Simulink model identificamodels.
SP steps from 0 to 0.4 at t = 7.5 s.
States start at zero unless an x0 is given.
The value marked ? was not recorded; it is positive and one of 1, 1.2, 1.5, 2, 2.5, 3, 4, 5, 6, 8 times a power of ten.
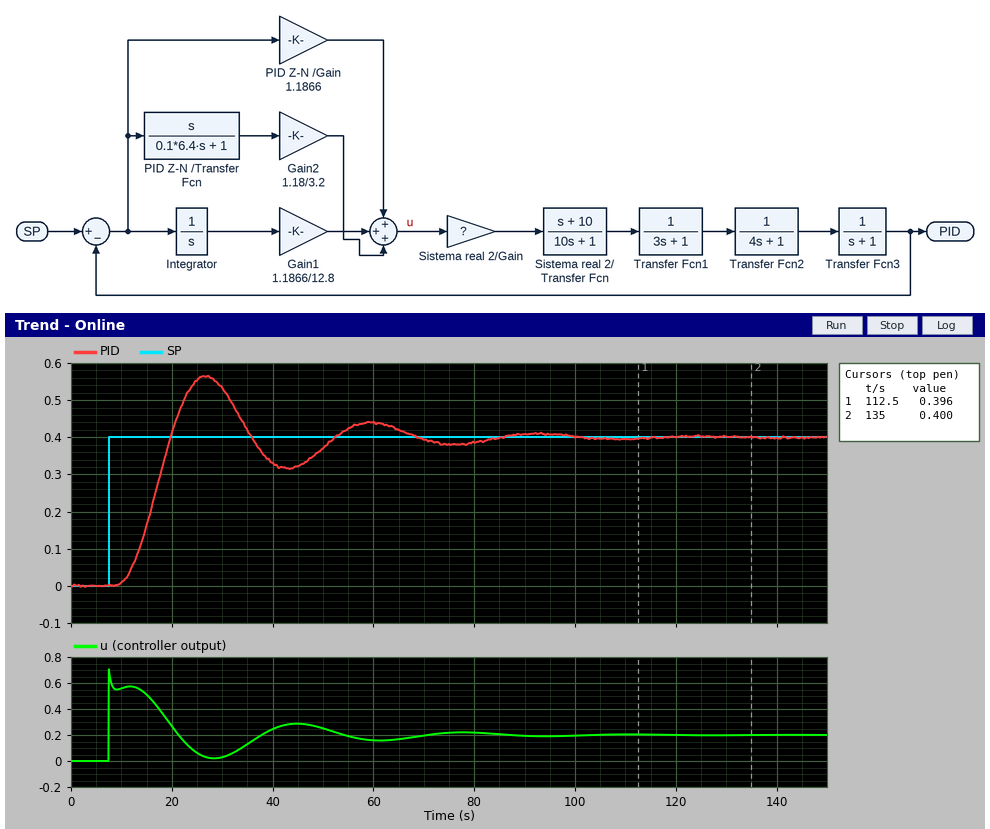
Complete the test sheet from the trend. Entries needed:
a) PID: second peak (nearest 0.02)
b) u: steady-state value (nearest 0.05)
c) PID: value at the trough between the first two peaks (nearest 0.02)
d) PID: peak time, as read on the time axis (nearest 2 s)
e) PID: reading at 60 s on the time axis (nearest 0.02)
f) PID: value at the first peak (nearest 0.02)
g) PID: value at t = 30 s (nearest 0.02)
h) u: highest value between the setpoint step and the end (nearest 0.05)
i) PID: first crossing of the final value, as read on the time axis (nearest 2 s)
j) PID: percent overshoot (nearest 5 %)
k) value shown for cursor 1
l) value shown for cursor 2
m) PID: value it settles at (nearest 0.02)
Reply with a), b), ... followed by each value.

a) 0.44
b) 0.20
c) 0.32
d) 26 s
e) 0.44
f) 0.56
g) 0.54
h) 0.70
i) 20 s
j) 40 %
k) 0.396
l) 0.400
m) 0.40
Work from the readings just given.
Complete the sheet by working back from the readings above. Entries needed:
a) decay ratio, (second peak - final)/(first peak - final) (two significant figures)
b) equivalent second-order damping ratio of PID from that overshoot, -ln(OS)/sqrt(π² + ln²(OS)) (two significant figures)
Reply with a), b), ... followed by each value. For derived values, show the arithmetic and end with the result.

a) (0.44 - 0.4) / (0.56 - 0.4) = 0.25
b) ln(0.4) = -0.916; 0.916 / sqrt(9.870 + 0.840) = 0.28
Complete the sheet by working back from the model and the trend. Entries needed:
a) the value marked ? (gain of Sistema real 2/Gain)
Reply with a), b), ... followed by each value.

a) 0.2
